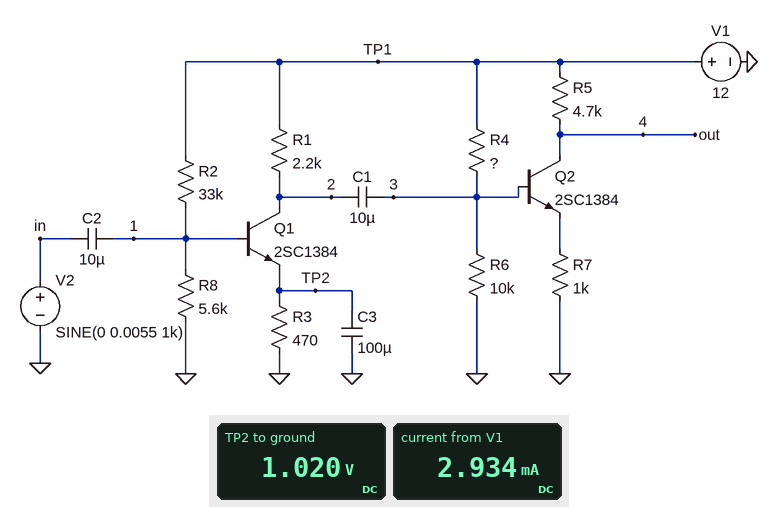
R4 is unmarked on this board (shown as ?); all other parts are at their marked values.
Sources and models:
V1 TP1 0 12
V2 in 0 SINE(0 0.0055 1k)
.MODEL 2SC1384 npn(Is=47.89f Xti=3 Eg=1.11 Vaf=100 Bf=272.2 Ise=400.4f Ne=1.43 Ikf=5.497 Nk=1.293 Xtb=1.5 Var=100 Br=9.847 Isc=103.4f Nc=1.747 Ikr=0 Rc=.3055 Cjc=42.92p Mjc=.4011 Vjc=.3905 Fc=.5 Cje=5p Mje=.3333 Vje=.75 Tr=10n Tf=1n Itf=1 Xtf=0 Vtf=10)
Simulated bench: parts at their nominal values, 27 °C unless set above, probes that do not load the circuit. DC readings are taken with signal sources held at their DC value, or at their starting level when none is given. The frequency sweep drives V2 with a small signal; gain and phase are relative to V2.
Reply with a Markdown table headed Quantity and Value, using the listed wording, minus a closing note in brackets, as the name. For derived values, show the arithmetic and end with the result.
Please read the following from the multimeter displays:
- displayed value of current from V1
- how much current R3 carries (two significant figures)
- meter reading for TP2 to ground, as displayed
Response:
| Quantity | Value |
|---|---|
| displayed value of current from V1 | 2.934 mA |
| how much current R3 carries | (1.02 V) / 470 Ω = 2.2 mA |
| meter reading for TP2 to ground, as displayed | 1.020 V |
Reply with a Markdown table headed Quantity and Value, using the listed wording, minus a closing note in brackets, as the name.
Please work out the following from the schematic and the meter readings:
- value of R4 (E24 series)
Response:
| Quantity | Value |
|---|---|
| value of R4 | 110 kΩ |
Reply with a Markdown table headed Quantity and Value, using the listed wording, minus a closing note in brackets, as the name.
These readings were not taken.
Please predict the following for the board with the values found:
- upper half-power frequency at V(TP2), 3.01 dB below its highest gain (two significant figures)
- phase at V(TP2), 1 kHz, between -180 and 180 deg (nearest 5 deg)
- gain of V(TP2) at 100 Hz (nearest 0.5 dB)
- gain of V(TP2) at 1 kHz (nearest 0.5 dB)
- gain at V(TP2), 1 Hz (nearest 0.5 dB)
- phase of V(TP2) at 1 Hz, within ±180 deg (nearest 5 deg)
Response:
| Quantity | Value |
|---|---|
| upper half-power frequency at V(TP2), 3.01 dB below its highest gain | 150 Hz |
| phase at V(TP2), 1 kHz, between -180 and 180 deg | -80 deg |
| gain of V(TP2) at 100 Hz | -2.5 dB |
| gain of V(TP2) at 1 kHz | -18.0 dB |
| gain at V(TP2), 1 Hz | -11.5 dB |
| phase of V(TP2) at 1 Hz, within ±180 deg | 75 deg |
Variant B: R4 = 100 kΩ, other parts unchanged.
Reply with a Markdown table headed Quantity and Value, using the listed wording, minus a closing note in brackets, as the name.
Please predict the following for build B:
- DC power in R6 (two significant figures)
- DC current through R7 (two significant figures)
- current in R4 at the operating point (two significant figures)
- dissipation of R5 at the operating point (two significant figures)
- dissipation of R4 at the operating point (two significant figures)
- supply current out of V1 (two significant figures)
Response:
| Quantity | Value |
|---|---|
| DC power in R6 | 110 µW |
| DC current through R7 | 450 µA |
| current in R4 at the operating point | 110 µA |
| dissipation of R5 at the operating point | 940 µW |
| dissipation of R4 at the operating point | 1.2 mW |
| supply current out of V1 | 3.0 mA |
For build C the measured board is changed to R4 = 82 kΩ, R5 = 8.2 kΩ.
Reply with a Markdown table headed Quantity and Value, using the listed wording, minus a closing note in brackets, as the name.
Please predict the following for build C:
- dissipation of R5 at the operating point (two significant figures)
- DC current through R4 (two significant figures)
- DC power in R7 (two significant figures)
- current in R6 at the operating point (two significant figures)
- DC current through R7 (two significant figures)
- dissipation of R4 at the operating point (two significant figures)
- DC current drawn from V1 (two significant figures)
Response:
| Quantity | Value |
|---|---|
| dissipation of R5 at the operating point | 3.3 mW |
| DC current through R4 | 130 µA |
| DC power in R7 | 410 µW |
| current in R6 at the operating point | 120 µA |
| DC current through R7 | 640 µA |
| dissipation of R4 at the operating point | 1.4 mW |
| DC current drawn from V1 | 3.2 mA |
